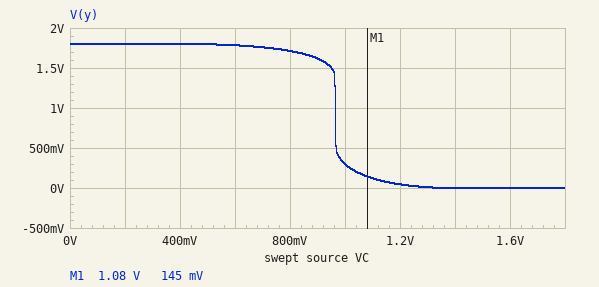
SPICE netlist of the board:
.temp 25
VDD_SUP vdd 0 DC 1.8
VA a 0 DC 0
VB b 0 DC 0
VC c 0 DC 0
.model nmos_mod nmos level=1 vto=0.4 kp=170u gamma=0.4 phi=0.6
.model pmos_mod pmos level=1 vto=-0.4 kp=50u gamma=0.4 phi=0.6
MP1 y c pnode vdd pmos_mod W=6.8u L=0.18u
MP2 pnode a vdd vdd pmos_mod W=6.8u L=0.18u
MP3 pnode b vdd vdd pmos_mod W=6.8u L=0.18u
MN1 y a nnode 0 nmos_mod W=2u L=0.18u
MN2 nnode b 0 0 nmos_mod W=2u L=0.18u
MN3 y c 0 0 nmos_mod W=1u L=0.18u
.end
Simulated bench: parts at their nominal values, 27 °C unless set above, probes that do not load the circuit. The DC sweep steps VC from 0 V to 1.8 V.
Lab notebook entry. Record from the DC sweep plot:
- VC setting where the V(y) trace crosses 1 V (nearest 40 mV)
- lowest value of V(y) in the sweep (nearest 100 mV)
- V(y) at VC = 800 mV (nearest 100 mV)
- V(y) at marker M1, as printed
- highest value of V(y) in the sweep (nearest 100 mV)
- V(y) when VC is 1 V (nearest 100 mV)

960 mV
0 V
1.7 V
145 mV
1.8 V
300 mV
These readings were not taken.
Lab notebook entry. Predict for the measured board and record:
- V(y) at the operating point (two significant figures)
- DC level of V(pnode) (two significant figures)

1.8 V
1.8 V
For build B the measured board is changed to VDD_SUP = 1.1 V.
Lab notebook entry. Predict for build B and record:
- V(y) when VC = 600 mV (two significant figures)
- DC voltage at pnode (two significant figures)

50 mV
1.1 V
